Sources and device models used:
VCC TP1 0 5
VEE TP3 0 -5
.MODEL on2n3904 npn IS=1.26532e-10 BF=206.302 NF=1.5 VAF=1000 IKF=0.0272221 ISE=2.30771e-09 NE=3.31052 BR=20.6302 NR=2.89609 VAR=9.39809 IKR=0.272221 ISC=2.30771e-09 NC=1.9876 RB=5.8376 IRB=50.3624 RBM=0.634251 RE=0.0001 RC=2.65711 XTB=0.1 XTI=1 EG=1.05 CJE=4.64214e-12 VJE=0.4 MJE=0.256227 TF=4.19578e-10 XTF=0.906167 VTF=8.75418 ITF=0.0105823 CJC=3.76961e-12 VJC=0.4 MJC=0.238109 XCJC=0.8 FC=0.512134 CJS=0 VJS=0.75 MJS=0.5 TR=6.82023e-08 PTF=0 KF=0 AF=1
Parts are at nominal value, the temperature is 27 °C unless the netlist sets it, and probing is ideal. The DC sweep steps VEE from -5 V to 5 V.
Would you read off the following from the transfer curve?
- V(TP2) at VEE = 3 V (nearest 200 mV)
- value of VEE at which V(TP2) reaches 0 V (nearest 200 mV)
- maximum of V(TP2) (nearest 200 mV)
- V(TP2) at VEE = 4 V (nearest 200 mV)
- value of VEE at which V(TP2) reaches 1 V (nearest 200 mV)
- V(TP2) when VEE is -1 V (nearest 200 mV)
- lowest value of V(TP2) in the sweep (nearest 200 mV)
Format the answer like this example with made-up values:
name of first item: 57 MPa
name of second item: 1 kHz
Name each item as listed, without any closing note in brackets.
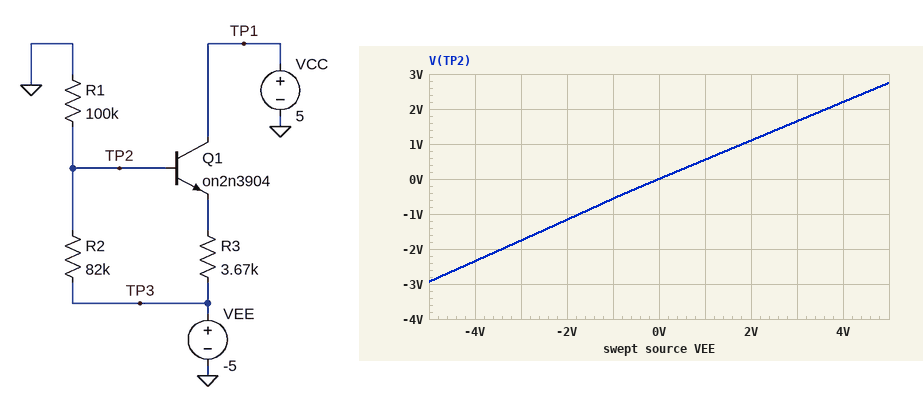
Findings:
V(TP2) at VEE = 3 V: 1.6 V
value of VEE at which V(TP2) reaches 0 V: 0 V
maximum of V(TP2): 2.8 V
V(TP2) at VEE = 4 V: 2.2 V
value of VEE at which V(TP2) reaches 1 V: 1.8 V
V(TP2) when VEE is -1 V: -600 mV
lowest value of V(TP2) in the sweep: -3.0 V
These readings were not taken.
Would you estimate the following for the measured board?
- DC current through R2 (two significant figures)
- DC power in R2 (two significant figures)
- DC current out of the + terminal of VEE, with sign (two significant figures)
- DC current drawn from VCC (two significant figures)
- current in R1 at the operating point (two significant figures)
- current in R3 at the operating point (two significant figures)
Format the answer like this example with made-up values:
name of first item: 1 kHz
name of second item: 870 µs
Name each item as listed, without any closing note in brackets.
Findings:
DC current through R2: 25 µA
DC power in R2: 52 µW
DC current out of the + terminal of VEE, with sign: -430 µA
DC current drawn from VCC: 400 µA
current in R1 at the operating point: 29 µA
current in R3 at the operating point: 400 µA
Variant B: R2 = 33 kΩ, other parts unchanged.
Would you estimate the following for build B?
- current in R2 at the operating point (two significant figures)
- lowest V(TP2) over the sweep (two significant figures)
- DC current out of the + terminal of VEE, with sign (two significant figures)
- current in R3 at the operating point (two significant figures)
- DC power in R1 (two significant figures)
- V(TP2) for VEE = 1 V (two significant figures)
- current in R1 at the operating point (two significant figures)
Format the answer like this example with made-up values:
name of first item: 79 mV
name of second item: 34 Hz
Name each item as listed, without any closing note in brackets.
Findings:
current in R2 at the operating point: 36 µA
lowest V(TP2) over the sweep: -3.8 V
DC current out of the + terminal of VEE, with sign: -210 µA
current in R3 at the operating point: 170 µA
DC power in R1: 150 µW
V(TP2) for VEE = 1 V: 750 mV
current in R1 at the operating point: 38 µA
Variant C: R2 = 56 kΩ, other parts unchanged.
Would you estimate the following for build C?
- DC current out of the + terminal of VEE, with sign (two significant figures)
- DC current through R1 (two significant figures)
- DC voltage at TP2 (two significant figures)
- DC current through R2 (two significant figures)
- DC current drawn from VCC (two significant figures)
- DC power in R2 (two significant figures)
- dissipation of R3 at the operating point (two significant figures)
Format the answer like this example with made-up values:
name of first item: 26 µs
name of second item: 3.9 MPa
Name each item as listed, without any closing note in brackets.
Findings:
DC current out of the + terminal of VEE, with sign: -330 µA
DC current through R1: 33 µA
DC voltage at TP2: -3.3 V
DC current through R2: 30 µA
DC current drawn from VCC: 300 µA
DC power in R2: 50 µW
dissipation of R3 at the operating point: 330 µW
